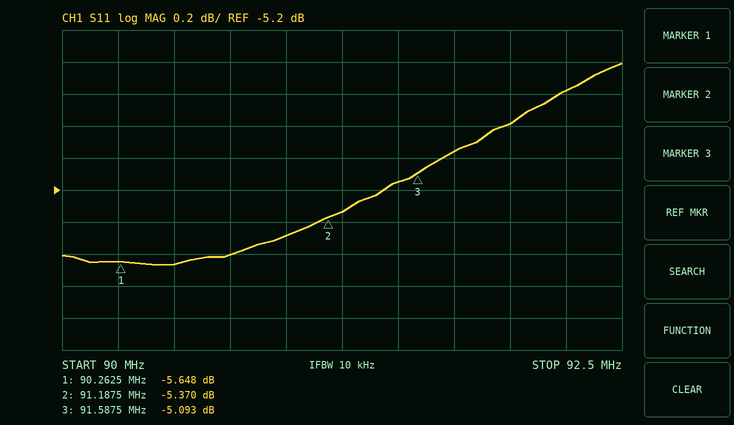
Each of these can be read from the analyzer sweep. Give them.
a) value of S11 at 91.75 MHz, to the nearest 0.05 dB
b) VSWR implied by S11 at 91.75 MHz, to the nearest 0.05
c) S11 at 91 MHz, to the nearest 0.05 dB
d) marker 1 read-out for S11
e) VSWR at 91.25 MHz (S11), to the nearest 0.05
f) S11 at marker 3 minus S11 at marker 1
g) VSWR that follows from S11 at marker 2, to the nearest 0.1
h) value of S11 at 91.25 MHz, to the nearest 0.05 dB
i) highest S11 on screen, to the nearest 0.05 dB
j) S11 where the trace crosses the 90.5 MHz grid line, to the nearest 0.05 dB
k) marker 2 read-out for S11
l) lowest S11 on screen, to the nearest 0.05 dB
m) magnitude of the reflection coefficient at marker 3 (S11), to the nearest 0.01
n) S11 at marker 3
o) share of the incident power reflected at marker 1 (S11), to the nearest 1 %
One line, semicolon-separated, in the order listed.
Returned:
-4.95 dB; 3.60; -5.50 dB; -5.648 dB; 3.35; 0.555 dB; 3.3; -5.35 dB; -4.40 dB; -5.65 dB; -5.370 dB; -5.65 dB; 0.56; -5.093 dB; 27 %
